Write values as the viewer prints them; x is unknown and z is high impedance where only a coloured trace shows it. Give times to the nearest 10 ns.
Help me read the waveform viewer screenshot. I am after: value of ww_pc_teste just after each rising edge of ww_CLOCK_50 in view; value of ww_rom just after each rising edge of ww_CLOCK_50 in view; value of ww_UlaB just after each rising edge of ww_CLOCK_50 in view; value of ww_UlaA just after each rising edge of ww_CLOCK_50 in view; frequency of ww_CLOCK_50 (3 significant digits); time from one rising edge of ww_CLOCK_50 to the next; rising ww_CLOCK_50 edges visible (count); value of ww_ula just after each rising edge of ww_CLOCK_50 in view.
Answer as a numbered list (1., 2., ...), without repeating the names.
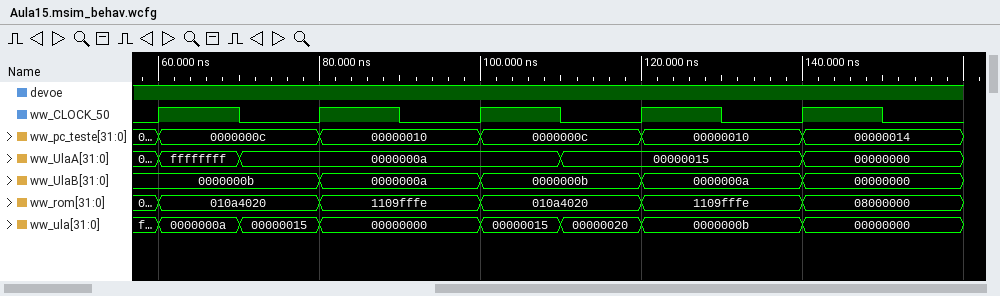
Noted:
1. 0000000c, 00000010, 0000000c, 00000010, 00000014
2. 010a4020, 1109fffe, 010a4020, 1109fffe, 08000000
3. 0000000b, 0000000a, 0000000b, 0000000a, 00000000
4. ffffffff, 0000000a, 0000000a, 00000015, 00000000
5. 50.0 MHz
6. 20 ns
7. 5
8. 0000000a, 00000000, 00000015, 0000000b, 00000000
